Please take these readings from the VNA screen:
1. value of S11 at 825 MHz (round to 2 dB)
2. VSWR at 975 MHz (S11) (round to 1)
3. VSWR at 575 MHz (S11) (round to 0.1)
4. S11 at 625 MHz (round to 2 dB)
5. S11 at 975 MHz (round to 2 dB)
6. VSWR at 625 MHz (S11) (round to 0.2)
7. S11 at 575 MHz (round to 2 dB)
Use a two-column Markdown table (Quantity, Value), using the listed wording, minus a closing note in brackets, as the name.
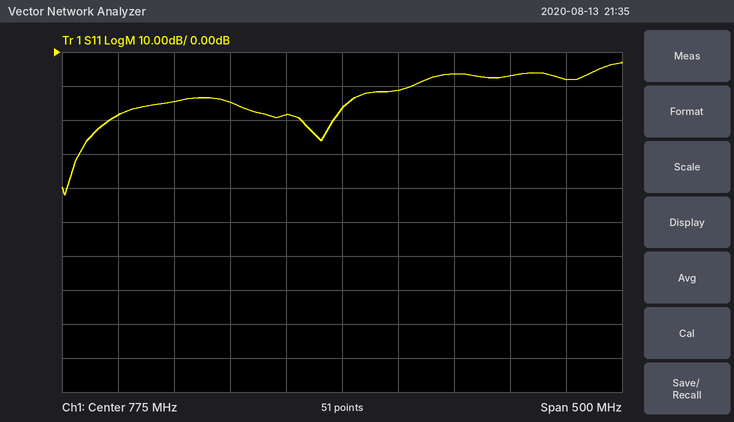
| Quantity | Value |
|---|---|
| value of S11 at 825 MHz | -12 dB |
| VSWR at 975 MHz (S11) | 2 |
| VSWR at 575 MHz (S11) | 1.3 |
| S11 at 625 MHz | -14 dB |
| S11 at 975 MHz | -8 dB |
| VSWR at 625 MHz (S11) | 1.4 |
| S11 at 575 MHz | -18 dB |
